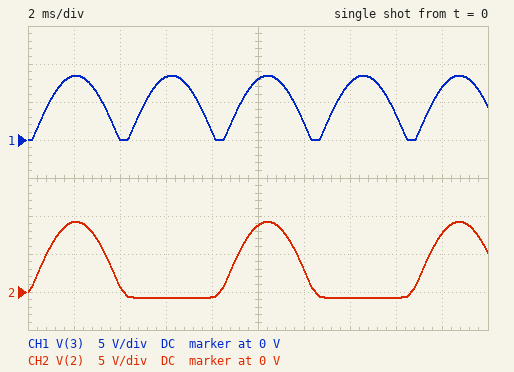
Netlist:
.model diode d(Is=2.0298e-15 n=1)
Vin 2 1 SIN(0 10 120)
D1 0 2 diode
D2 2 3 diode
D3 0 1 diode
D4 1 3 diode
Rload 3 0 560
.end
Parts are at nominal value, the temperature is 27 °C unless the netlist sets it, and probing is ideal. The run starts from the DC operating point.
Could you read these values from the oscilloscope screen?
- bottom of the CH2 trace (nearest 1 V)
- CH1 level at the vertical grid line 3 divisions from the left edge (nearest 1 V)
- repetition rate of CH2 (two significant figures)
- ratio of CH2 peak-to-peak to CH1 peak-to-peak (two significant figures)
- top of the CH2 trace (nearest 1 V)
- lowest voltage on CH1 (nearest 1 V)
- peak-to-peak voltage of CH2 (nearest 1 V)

-1 V
8 V
120 Hz
1.2
9 V
0 V
10 V
